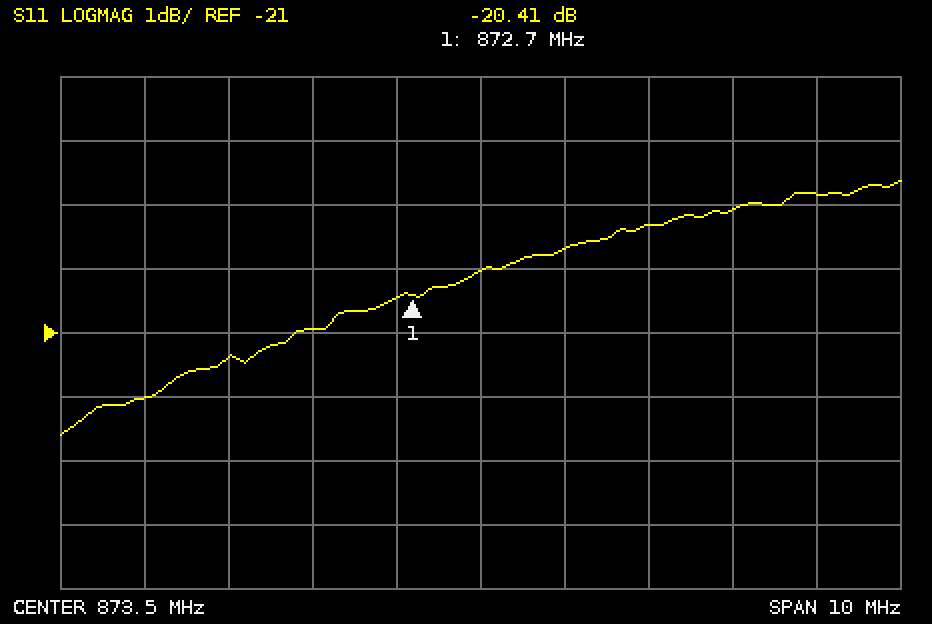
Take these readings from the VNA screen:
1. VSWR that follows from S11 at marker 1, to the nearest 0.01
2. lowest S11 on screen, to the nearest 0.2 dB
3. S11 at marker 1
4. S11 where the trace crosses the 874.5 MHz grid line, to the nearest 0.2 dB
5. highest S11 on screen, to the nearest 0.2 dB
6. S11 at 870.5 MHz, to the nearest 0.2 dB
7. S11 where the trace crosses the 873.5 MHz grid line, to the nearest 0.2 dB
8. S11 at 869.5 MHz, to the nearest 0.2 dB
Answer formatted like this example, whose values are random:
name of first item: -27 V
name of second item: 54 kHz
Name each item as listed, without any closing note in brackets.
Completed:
VSWR that follows from S11 at marker 1, to the nearest 0.01: 1.21
lowest S11 on screen, to the nearest 0.2 dB: -22.6 dB
S11 at marker 1: -20.41 dB
S11 where the trace crosses the 874.5 MHz grid line, to the nearest 0.2 dB: -19.6 dB
highest S11 on screen, to the nearest 0.2 dB: -18.6 dB
S11 at 870.5 MHz, to the nearest 0.2 dB: -21.4 dB
S11 where the trace crosses the 873.5 MHz grid line, to the nearest 0.2 dB: -20.0 dB
S11 at 869.5 MHz, to the nearest 0.2 dB: -22.0 dB
